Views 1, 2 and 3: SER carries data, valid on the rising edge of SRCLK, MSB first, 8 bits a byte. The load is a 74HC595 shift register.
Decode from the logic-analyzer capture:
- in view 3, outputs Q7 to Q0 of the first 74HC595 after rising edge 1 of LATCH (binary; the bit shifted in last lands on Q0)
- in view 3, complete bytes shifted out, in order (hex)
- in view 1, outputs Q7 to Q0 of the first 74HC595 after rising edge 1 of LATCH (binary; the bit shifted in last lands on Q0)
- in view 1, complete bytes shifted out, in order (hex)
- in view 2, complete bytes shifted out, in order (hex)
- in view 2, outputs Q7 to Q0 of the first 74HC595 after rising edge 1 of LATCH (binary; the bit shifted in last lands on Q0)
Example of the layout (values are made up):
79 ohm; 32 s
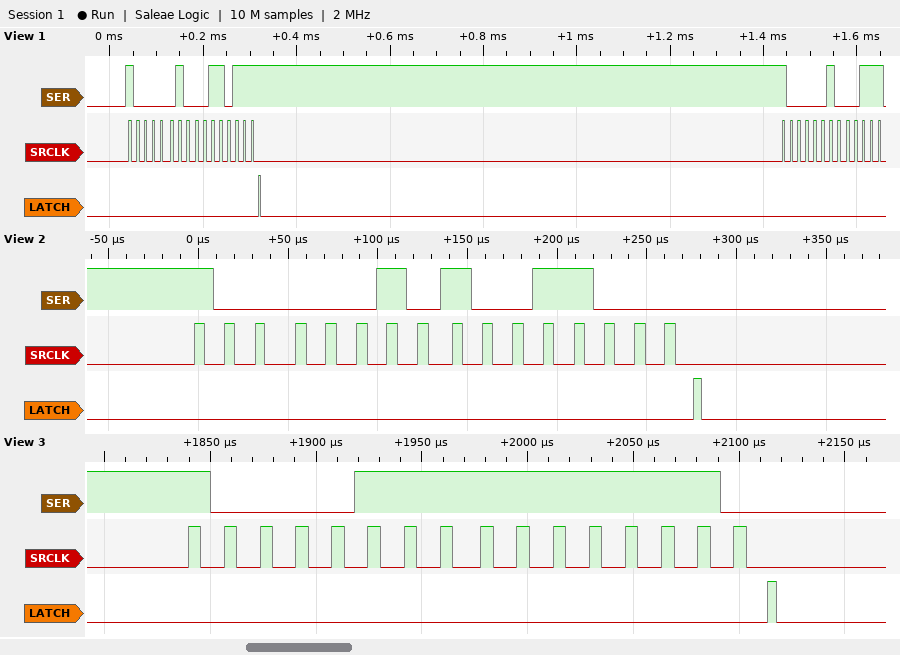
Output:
11111110; 87 FE; 00110111; 0x82 0x37 0x82; 0x82 0x98; 10011000
